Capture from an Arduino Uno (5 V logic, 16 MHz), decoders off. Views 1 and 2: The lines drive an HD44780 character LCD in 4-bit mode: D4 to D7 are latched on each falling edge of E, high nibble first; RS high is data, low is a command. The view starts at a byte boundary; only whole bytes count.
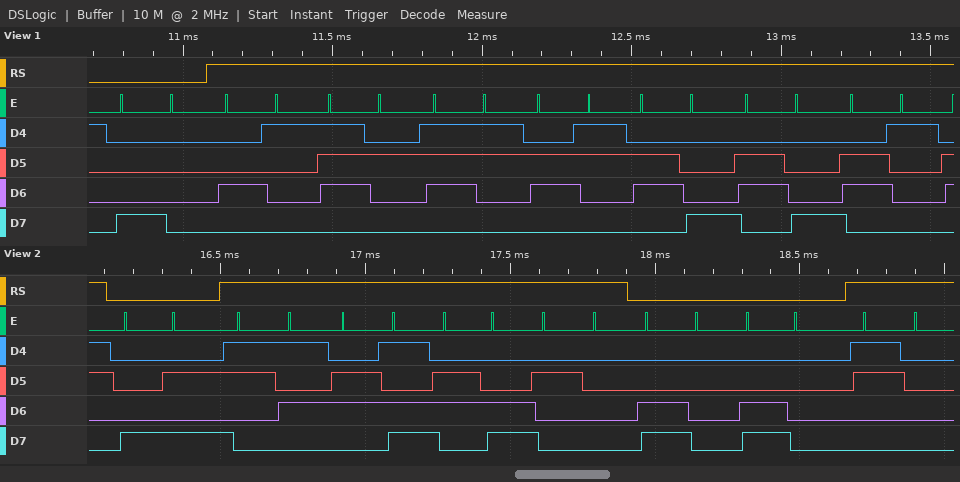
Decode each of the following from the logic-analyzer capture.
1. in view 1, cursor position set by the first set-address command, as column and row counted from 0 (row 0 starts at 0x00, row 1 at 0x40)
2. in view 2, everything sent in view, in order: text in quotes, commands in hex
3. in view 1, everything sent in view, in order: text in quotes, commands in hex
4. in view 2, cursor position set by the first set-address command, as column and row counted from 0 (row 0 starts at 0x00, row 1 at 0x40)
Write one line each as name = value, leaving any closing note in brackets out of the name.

in view 1, cursor position set by the first set-address command, as column and row counted from 0 = column 0, row 0
in view 2, everything sent in view, in order: text in quotes, commands in hex = 0x8A "5ml " 0xC0 0xC0 "0"
in view 1, everything sent in view, in order: text in quotes, commands in hex = 0x80 "Arschha"
in view 2, cursor position set by the first set-address command, as column and row counted from 0 = column 10, row 0
